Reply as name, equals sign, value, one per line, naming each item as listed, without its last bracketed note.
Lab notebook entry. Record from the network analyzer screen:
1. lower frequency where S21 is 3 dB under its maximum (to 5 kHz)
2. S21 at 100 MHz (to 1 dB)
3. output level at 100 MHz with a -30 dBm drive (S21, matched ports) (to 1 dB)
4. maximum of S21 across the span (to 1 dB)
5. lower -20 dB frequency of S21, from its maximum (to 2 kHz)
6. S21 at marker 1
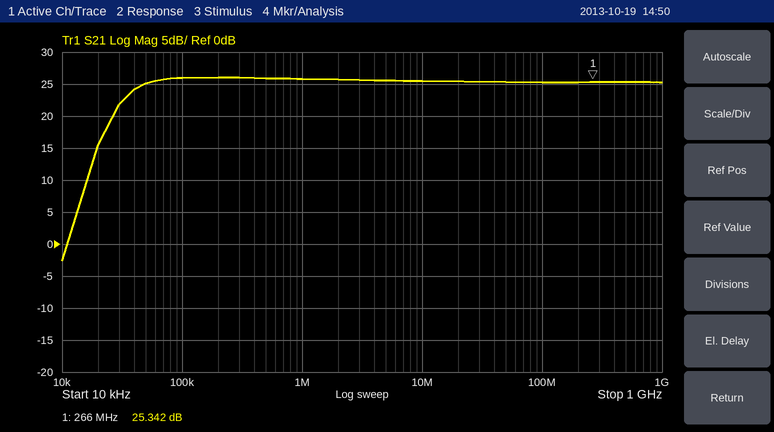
lower frequency where S21 is 3 dB under its maximum = 35 kHz
S21 at 100 MHz = 25 dB
output level at 100 MHz with a -30 dBm drive (S21, matched ports) = -5 dBm
maximum of S21 across the span = 26 dB
lower -20 dB frequency of S21, from its maximum = 14 kHz
S21 at marker 1 = 25.342 dB
